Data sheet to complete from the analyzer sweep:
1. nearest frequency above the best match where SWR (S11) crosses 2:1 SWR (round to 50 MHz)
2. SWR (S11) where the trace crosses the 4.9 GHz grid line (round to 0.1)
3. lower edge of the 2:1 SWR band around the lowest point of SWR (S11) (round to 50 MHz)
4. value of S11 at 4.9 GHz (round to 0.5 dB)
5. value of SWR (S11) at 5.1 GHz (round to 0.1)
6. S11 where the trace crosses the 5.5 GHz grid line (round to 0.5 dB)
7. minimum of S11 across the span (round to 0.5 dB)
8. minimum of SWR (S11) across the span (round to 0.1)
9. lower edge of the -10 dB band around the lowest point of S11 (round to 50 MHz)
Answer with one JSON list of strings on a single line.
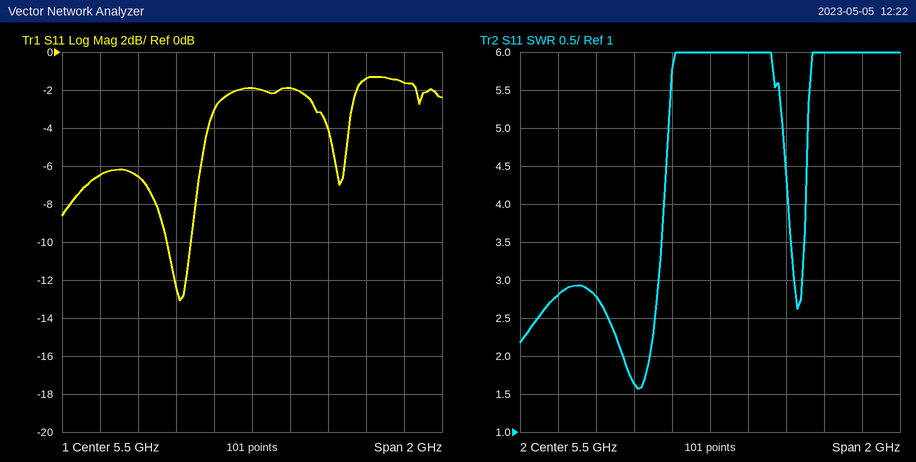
["5.20 GHz", "2.8", "5.05 GHz", "-6.5 dB", "1.6", "-2.0 dB", "-13.0 dB", "1.6", "5.05 GHz"]
